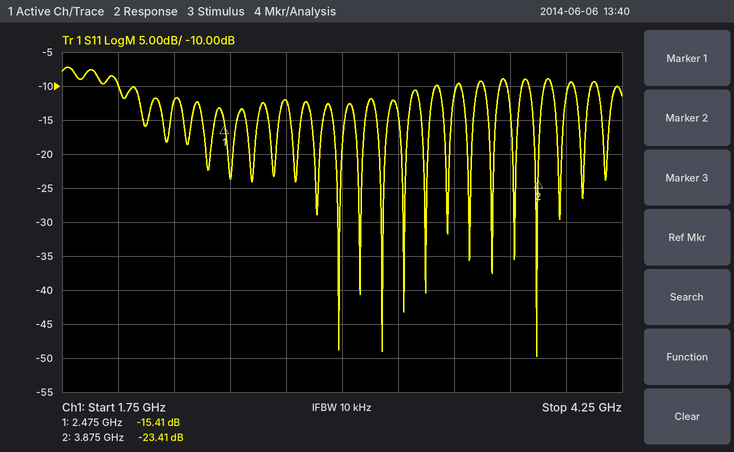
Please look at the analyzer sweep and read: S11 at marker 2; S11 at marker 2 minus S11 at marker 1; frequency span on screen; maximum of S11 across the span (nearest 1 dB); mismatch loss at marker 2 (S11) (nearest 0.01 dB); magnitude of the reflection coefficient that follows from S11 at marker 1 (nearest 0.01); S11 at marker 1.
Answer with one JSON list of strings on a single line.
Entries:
["-23.41 dB", "-8.00 dB", "2.5 GHz", "-7 dB", "0.02 dB", "0.17", "-15.41 dB"]
